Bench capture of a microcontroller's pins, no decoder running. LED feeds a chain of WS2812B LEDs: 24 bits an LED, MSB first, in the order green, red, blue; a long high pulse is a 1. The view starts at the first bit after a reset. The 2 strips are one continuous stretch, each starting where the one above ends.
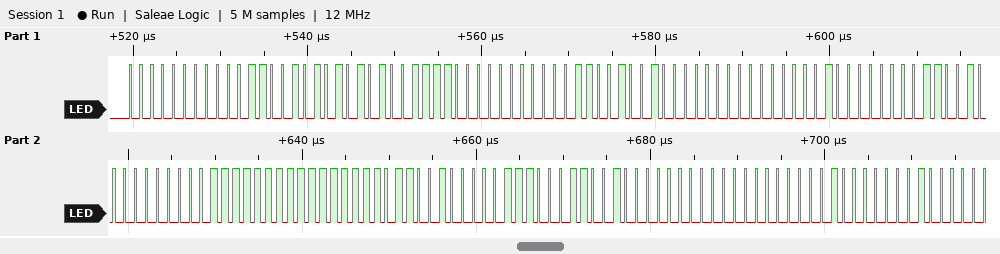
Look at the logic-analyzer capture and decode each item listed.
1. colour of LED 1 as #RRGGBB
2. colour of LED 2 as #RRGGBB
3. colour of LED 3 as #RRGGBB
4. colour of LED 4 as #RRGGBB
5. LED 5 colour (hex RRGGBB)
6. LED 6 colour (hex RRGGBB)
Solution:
#190055
#003C64
#008080
#0064FF
#64FF1C
#006400
